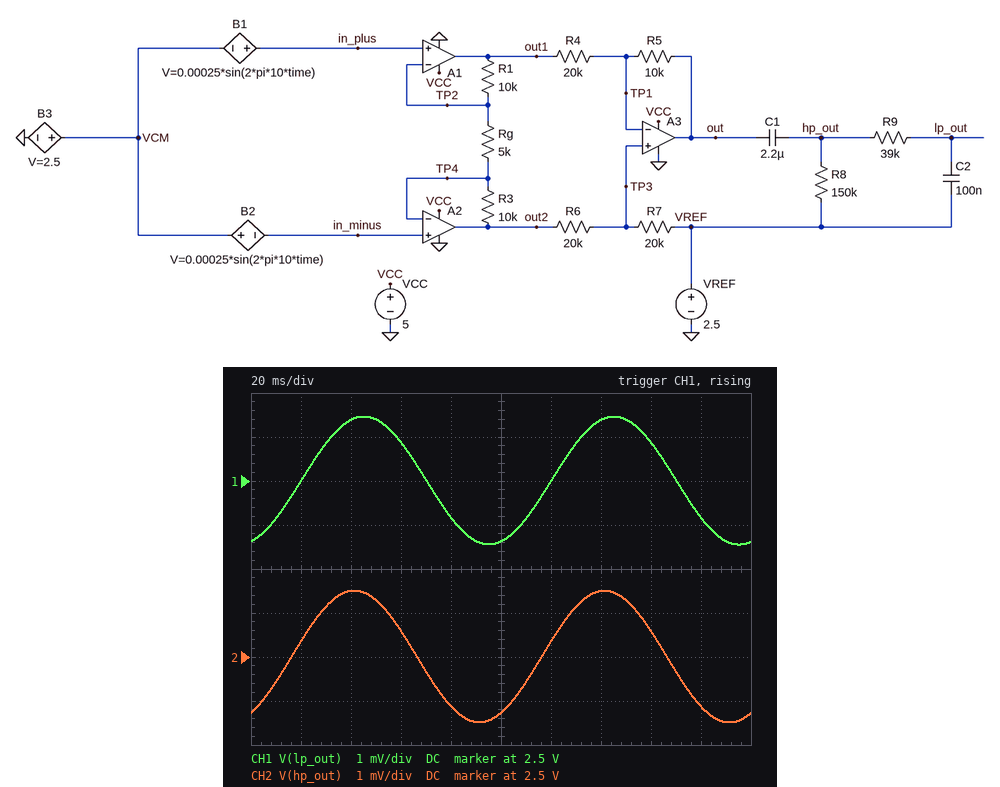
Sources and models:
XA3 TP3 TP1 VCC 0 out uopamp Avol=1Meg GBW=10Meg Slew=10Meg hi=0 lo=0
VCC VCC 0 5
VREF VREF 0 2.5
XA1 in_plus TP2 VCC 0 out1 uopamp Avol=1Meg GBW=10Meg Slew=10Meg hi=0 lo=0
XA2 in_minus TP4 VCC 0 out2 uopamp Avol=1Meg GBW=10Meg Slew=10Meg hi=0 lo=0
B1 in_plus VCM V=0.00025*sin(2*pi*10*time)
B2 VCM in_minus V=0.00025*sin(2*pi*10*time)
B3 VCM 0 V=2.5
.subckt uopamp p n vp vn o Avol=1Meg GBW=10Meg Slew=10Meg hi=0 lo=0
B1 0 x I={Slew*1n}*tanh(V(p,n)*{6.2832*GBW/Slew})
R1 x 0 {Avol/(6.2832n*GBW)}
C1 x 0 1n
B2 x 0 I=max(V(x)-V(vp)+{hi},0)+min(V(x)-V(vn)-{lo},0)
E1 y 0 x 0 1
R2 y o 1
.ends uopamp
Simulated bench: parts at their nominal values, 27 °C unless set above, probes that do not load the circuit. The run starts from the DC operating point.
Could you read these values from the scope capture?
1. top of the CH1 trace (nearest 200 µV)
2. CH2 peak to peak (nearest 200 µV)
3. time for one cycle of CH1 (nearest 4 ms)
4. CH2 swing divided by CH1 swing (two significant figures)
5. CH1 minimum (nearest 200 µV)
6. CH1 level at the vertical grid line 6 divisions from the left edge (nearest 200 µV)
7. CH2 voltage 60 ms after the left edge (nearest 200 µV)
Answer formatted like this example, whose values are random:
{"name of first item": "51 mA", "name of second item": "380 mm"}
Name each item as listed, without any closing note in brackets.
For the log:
{"top of the CH1 trace": "2.5014 V", "CH2 peak to peak": "3.0 mV", "time for one cycle of CH1": "100 ms", "CH2 swing divided by CH1 swing": "1.0", "CH1 minimum": "2.4986 V", "CH1 level at the vertical grid line 6 divisions from the left edge": "2.5000 V", "CH2 voltage 60 ms after the left edge": "2.5006 V"}
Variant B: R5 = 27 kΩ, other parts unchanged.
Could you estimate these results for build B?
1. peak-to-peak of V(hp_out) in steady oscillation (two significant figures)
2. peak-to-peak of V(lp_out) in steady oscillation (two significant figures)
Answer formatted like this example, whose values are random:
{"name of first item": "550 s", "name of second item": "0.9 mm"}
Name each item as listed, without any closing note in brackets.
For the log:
{"peak-to-peak of V(hp_out) in steady oscillation": "6.1 mV", "peak-to-peak of V(lp_out) in steady oscillation": "5.9 mV"}
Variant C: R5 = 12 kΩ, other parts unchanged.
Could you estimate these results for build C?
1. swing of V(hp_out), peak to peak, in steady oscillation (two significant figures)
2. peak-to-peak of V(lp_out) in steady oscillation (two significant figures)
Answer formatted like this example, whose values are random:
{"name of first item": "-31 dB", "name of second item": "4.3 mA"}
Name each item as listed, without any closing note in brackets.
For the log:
{"swing of V(hp_out), peak to peak, in steady oscillation": "3.4 mV", "peak-to-peak of V(lp_out) in steady oscillation": "3.3 mV"}
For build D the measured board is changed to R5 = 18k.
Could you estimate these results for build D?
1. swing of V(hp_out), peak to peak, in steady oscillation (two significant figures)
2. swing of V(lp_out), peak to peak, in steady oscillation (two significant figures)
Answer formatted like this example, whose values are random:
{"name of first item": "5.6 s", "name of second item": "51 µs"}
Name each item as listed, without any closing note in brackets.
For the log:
{"swing of V(hp_out), peak to peak, in steady oscillation": "4.4 mV", "swing of V(lp_out), peak to peak, in steady oscillation": "4.3 mV"}
